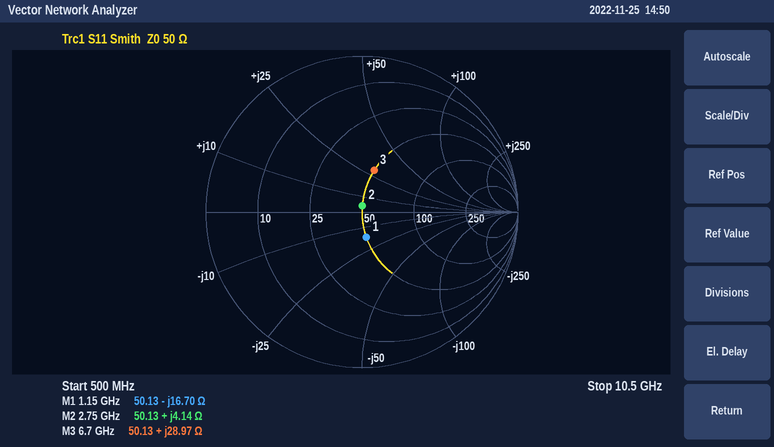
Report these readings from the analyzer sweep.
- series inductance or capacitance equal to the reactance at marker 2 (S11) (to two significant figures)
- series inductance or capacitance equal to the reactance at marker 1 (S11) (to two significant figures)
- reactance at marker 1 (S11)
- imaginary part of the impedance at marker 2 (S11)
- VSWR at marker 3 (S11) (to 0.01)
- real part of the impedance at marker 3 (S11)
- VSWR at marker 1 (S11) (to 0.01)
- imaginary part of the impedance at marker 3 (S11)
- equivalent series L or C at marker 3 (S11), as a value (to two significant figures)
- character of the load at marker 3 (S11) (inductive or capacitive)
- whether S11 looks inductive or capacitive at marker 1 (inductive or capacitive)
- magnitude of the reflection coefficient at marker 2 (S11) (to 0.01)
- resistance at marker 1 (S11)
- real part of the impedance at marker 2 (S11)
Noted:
240 pH
8.3 pF
-16.70 Ω
+4.14 Ω
1.77
50.13 Ω
1.39
+28.97 Ω
690 pH
inductive
capacitive
0.04
50.13 Ω
50.13 Ω
